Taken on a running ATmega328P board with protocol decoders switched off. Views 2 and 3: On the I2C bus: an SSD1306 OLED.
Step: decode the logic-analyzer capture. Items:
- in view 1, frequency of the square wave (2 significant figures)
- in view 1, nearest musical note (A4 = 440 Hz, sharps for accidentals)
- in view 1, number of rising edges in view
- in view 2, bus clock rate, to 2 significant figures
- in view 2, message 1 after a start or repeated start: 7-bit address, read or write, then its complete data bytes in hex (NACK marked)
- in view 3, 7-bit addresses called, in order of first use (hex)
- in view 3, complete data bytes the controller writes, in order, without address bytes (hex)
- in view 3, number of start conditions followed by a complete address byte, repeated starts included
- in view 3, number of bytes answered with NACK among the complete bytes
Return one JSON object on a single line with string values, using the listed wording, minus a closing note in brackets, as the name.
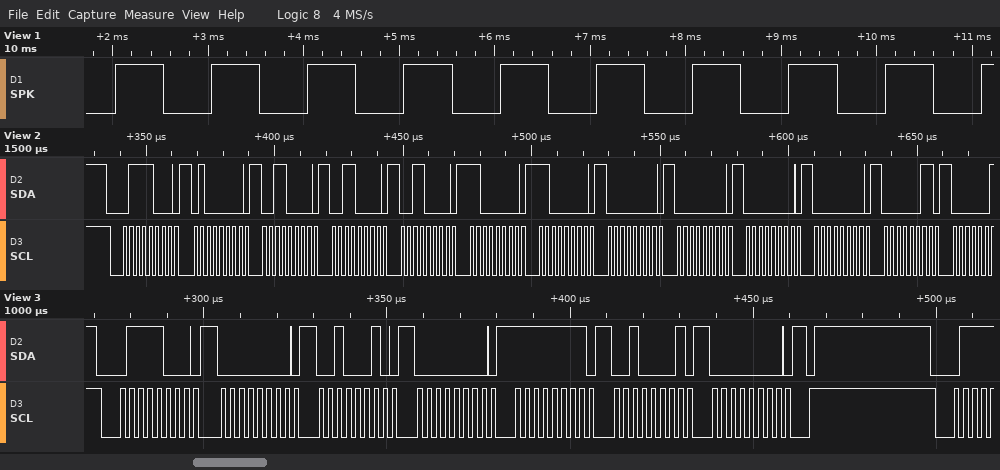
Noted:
{"in view 1, frequency of the square wave": "990 Hz", "in view 1, nearest musical note": "B5", "in view 1, number of rising edges in view": "10", "in view 2, bus clock rate, to 2 significant figures": "400 kHz", "in view 2, message 1 after a start or repeated start: 7-bit address, read or write, then its complete data bytes in hex": "0x3C write: 40 30 30 30 C0 C0 00 00 00 00 03", "in view 3, 7-bit addresses called, in order of first use": "0x3C", "in view 3, complete data bytes the controller writes, in order, without address bytes": "00 22 00 FF 21 00", "in view 3, number of start conditions followed by a complete address byte, repeated starts included": "1", "in view 3, number of bytes answered with NACK among the complete bytes": "0"}
